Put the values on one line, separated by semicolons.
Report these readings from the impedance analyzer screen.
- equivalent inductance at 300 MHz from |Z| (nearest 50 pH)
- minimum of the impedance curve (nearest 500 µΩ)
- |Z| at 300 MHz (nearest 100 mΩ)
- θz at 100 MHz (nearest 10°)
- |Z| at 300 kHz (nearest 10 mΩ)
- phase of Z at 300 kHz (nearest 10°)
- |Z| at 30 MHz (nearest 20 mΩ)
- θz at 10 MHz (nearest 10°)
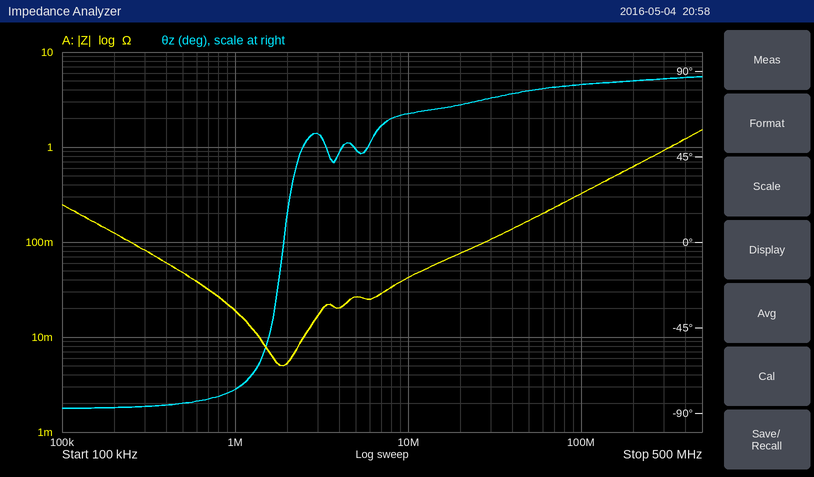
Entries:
500 pH; 5.0 mΩ; 900 mΩ; 80°; 80 mΩ; -90°; 100 mΩ; 70°
